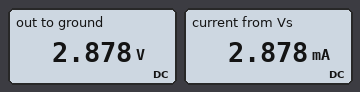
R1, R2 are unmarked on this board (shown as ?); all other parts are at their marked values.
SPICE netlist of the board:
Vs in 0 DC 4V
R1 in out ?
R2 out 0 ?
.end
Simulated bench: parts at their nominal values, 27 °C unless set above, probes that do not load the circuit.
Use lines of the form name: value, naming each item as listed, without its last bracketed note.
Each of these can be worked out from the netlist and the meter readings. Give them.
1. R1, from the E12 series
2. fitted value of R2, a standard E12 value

R1, from the E12 series: 390 Ω
fitted value of R2, a standard E12 value: 1 kΩ
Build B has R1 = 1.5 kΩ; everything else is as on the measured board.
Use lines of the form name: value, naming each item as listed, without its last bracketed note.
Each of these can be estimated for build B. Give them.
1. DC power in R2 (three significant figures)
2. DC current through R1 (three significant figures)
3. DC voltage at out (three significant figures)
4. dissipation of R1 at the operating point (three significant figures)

DC power in R2: 2.56 mW
DC current through R1: 1.60 mA
DC voltage at out: 1.60 V
dissipation of R1 at the operating point: 3.84 mW
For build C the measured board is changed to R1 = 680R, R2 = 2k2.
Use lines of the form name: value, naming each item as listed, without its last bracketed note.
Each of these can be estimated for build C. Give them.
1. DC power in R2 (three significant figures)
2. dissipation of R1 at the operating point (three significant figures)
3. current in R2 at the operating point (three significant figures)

DC power in R2: 4.24 mW
dissipation of R1 at the operating point: 1.31 mW
current in R2 at the operating point: 1.39 mA
